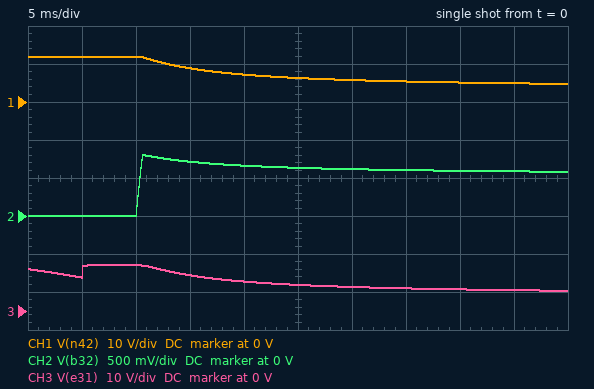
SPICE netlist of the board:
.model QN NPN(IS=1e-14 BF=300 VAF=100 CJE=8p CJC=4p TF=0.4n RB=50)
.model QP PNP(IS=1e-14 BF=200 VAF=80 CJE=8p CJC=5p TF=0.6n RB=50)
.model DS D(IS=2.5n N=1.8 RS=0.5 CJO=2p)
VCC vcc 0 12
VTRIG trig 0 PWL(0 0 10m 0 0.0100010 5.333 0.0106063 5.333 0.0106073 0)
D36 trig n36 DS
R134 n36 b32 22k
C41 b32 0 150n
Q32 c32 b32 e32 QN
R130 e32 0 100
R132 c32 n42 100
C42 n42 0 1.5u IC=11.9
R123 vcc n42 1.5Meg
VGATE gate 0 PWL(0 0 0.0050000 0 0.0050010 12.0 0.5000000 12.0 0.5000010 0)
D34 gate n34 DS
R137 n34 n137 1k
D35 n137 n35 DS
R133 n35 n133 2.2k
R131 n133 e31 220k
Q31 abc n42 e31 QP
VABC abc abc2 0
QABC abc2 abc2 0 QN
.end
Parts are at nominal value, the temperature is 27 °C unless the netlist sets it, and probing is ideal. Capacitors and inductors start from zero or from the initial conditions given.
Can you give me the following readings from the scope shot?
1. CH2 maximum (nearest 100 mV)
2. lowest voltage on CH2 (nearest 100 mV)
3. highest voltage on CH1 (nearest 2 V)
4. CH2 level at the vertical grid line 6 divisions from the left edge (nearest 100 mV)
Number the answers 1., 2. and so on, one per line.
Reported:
1. 800 mV
2. 0 V
3. 12 V
4. 600 mV
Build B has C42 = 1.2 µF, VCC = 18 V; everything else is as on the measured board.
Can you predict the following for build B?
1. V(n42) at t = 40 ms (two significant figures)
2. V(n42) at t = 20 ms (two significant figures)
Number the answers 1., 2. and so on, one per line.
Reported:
1. 3.6 V
2. 6.1 V
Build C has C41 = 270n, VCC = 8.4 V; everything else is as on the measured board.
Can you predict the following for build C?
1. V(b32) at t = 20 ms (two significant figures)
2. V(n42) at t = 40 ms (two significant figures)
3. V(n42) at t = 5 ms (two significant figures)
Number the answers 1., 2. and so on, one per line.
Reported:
1. 470 mV
2. 12 V
3. 12 V
